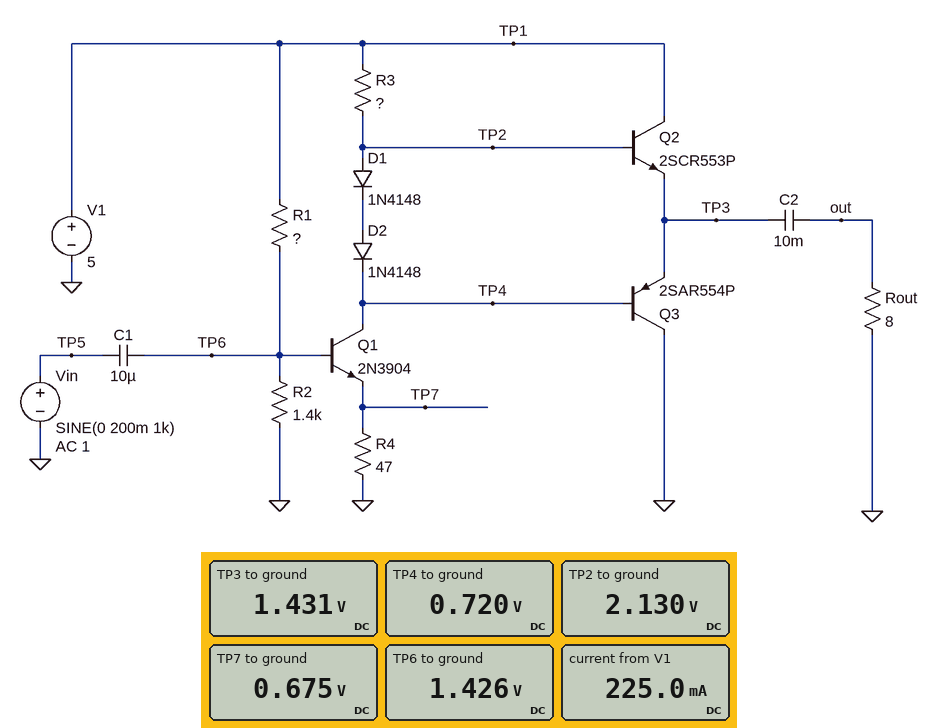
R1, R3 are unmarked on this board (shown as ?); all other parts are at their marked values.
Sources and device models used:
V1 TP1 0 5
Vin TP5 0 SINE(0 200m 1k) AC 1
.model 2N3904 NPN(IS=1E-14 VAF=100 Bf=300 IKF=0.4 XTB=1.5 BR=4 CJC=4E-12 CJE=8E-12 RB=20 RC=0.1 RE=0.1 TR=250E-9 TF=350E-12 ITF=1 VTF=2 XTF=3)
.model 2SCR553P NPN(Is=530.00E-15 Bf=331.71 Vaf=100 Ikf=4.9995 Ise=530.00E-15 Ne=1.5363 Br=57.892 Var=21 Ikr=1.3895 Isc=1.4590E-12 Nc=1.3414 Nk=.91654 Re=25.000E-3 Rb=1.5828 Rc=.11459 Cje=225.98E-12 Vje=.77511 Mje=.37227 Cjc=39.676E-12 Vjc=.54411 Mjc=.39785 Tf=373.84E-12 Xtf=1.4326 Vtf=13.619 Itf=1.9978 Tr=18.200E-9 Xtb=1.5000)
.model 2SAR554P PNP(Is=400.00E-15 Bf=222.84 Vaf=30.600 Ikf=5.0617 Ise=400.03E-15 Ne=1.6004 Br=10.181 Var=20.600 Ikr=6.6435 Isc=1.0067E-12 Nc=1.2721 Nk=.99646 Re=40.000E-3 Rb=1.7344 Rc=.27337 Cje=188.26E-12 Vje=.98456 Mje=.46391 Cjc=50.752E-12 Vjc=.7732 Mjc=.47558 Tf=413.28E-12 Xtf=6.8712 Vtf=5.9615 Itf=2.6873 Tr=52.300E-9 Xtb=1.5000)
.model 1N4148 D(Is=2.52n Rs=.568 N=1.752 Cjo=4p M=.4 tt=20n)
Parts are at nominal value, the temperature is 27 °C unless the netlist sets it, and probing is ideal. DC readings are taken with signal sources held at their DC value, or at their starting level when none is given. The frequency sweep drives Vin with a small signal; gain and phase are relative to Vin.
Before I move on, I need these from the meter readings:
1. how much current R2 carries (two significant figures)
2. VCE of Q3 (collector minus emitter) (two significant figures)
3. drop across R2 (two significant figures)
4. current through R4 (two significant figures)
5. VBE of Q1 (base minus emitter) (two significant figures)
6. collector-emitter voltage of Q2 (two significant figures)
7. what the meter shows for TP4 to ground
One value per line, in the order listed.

1.0 mA
-1.4 V
1.4 V
14 mA
750 mV
3.6 V
0.720 V
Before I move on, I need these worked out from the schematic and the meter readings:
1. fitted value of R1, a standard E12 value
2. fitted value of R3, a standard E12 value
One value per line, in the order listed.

1.8 kΩ
220 Ω
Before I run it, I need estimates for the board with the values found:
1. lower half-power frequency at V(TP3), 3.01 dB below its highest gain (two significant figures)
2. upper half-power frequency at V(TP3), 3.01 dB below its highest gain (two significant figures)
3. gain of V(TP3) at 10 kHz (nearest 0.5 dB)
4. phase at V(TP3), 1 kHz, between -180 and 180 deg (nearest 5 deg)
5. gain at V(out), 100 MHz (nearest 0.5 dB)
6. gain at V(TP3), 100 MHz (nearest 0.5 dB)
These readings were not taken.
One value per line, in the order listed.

140 kHz
88 MHz
-10.5 dB
15 deg
-7.5 dB
-7.5 dB
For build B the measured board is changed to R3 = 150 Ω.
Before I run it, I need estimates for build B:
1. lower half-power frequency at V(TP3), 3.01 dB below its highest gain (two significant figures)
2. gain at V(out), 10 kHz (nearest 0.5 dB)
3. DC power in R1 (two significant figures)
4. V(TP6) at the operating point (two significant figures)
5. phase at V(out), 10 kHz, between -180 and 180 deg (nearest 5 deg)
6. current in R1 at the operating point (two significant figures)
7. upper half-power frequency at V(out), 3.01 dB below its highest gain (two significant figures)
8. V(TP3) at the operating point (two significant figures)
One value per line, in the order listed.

190 kHz
-17.5 dB
6.3 mW
1.6 V
10 deg
1.9 mA
88 MHz
1.7 V
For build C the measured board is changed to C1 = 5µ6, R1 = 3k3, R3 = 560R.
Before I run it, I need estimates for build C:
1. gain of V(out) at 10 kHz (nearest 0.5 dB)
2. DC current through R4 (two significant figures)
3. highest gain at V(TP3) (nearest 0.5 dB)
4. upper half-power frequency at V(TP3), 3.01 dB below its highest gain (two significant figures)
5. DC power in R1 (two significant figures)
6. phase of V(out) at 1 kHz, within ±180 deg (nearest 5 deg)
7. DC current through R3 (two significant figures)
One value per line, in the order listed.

-24.0 dB
6.5 mA
-3.5 dB
77 MHz
4.8 mW
25 deg
5.9 mA
